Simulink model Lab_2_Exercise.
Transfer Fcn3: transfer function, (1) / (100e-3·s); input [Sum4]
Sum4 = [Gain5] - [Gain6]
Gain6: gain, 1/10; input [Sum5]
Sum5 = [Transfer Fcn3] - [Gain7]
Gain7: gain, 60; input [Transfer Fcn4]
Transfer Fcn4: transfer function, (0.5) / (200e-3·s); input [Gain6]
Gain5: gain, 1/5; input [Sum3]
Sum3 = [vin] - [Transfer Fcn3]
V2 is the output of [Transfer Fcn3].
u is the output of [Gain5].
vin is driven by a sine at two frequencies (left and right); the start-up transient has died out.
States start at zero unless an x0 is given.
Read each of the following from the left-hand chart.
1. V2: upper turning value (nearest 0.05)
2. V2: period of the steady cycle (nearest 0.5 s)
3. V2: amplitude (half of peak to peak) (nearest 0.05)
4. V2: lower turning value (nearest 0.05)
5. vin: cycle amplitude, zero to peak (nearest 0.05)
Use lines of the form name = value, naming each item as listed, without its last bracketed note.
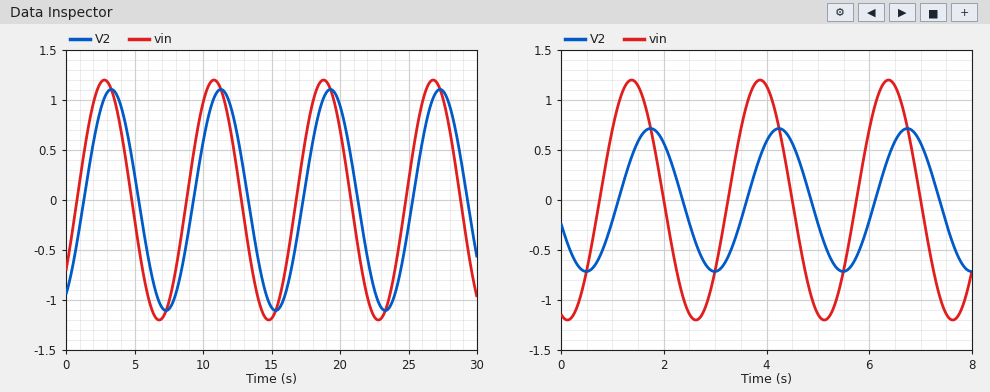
V2: upper turning value = 1.10
V2: period of the steady cycle = 8.0 s
V2: amplitude (half of peak to peak) = 1.10
V2: lower turning value = -1.10
vin: cycle amplitude, zero to peak = 1.20
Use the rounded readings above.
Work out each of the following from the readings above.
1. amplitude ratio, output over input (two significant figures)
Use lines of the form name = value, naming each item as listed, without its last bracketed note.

amplitude ratio, output over input = 0.92
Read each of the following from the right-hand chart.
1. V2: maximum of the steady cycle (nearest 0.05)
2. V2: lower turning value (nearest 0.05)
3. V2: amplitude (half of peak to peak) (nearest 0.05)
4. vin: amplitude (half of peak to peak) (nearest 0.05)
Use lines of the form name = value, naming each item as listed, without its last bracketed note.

V2: maximum of the steady cycle = 0.70
V2: lower turning value = -0.70
V2: amplitude (half of peak to peak) = 0.70
vin: amplitude (half of peak to peak) = 1.20
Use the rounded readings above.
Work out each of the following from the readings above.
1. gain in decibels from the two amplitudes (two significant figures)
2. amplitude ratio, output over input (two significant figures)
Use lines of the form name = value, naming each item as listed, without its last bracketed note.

gain in decibels from the two amplitudes = -4.7 dB
amplitude ratio, output over input = 0.58
